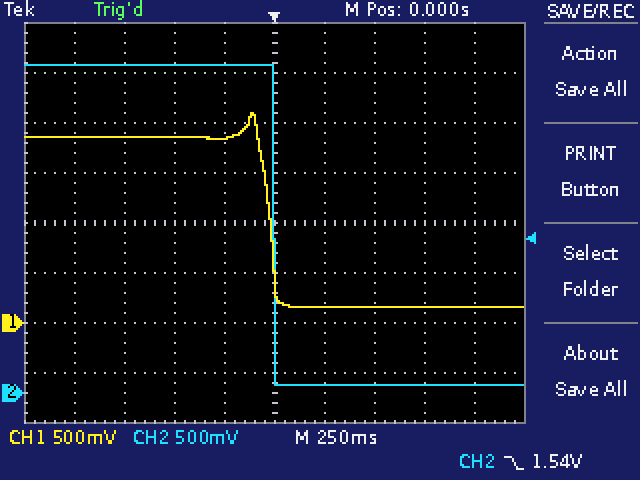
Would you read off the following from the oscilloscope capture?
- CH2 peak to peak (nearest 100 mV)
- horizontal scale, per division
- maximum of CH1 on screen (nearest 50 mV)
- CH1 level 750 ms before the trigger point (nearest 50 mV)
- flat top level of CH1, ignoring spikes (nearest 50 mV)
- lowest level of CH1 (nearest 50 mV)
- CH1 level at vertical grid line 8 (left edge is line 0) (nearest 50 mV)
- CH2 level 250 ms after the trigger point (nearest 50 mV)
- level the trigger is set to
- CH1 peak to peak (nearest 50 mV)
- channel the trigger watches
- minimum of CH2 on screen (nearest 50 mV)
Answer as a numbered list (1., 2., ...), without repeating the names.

1. 3.20 V
2. 250 ms
3. 2.10 V
4. 1.85 V
5. 1.85 V
6. 150 mV
7. 150 mV
8. 100 mV
9. 1.54 V
10. 1.95 V
11. CH2
12. 100 mV
